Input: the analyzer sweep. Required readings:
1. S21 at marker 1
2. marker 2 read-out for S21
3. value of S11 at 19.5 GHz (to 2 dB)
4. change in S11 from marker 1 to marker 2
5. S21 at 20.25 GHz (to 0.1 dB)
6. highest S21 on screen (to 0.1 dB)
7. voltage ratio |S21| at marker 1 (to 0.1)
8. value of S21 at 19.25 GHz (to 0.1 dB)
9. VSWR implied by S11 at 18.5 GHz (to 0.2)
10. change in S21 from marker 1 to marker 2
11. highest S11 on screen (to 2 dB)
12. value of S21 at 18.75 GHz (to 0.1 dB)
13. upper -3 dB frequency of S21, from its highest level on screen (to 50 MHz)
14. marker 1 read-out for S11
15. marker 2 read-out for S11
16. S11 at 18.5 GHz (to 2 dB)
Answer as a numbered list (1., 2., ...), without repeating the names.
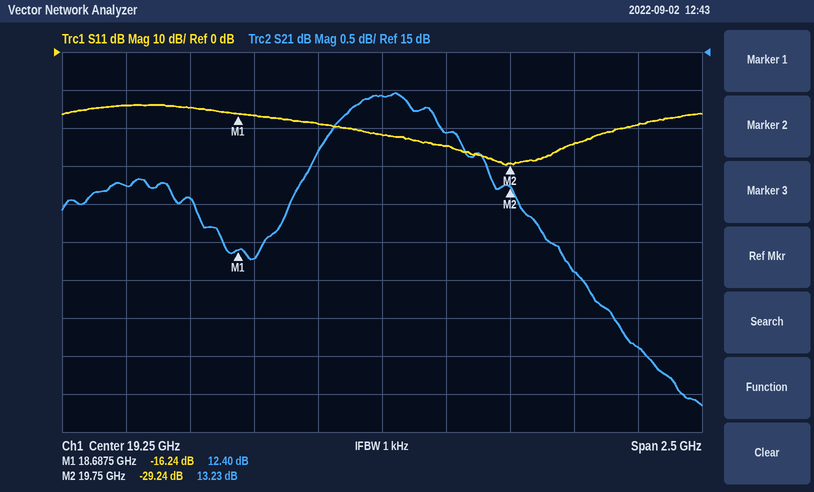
1. 12.40 dB
2. 13.23 dB
3. -24 dB
4. -13.00 dB
5. 11.1 dB
6. 14.5 dB
7. 4.2
8. 14.4 dB
9. 1.4
10. 0.83 dB
11. -14 dB
12. 12.3 dB
13. 20.15 GHz
14. -16.24 dB
15. -29.24 dB
16. -14 dB
